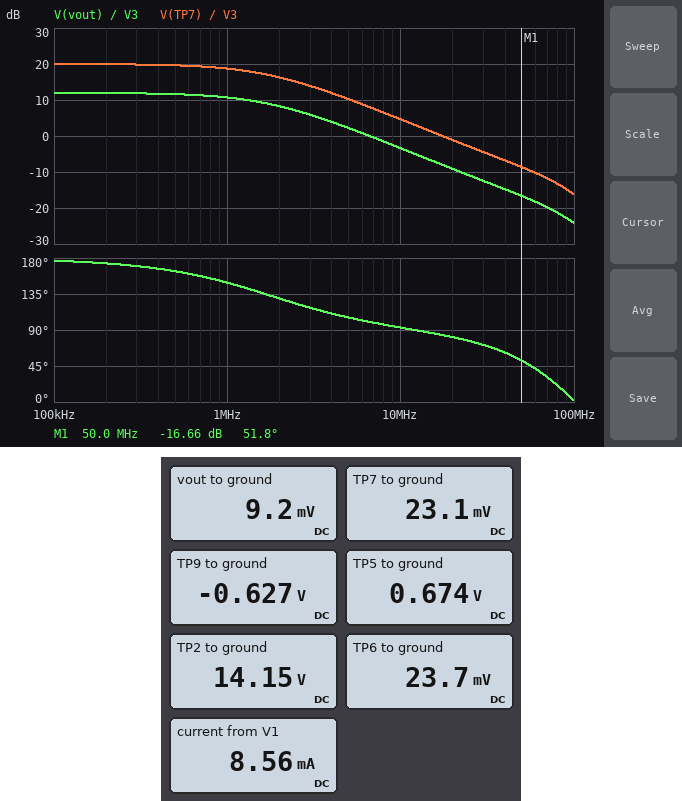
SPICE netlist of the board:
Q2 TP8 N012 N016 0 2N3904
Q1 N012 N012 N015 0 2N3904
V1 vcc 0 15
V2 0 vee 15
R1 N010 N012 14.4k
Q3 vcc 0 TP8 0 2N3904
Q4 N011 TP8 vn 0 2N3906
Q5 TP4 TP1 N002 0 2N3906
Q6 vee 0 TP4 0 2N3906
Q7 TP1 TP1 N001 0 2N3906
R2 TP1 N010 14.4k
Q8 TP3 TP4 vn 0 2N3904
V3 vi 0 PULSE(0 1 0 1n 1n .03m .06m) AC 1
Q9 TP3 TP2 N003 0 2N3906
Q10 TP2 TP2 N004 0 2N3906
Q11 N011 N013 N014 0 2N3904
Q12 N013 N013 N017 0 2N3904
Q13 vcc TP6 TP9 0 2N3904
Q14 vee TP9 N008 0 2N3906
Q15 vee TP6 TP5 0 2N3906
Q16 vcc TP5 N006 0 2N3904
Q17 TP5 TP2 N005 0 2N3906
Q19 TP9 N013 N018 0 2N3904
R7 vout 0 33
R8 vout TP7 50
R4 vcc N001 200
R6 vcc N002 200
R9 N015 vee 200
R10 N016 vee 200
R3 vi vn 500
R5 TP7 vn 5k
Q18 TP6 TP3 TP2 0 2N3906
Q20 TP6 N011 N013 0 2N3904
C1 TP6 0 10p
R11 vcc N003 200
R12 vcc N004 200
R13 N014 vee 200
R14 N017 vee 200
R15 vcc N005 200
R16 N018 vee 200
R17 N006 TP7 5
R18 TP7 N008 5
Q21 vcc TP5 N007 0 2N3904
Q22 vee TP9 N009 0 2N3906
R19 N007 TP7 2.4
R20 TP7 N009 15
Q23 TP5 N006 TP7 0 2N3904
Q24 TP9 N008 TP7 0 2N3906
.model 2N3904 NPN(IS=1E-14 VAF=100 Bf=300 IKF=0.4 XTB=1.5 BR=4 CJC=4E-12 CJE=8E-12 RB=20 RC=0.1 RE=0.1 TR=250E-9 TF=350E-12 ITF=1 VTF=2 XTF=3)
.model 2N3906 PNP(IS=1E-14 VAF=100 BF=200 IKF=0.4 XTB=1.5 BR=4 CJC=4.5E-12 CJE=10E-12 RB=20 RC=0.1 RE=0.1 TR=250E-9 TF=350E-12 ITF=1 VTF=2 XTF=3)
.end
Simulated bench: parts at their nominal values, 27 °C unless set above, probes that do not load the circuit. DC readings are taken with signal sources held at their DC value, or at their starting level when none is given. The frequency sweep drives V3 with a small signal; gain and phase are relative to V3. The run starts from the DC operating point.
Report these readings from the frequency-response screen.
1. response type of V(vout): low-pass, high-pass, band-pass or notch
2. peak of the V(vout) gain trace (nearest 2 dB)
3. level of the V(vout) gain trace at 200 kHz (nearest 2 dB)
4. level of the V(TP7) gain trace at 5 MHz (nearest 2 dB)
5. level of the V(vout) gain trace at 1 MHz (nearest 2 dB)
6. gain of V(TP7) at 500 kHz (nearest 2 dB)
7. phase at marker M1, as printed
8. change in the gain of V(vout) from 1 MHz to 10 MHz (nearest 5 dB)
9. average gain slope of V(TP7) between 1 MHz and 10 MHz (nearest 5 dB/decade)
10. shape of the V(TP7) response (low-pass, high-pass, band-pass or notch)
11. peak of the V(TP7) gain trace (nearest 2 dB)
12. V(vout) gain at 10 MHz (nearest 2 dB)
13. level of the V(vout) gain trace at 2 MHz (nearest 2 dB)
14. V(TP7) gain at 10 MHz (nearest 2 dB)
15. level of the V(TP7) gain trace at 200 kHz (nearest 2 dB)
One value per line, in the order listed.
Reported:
low-pass
12 dB
12 dB
10 dB
10 dB
20 dB
51.8 deg
-15 dB
-15 dB/decade
low-pass
20 dB
-4 dB
8 dB
4 dB
20 dB
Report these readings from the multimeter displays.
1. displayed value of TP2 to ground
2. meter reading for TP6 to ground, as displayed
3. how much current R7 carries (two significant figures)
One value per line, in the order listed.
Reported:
14.15 V
23.7 mV
280 µA
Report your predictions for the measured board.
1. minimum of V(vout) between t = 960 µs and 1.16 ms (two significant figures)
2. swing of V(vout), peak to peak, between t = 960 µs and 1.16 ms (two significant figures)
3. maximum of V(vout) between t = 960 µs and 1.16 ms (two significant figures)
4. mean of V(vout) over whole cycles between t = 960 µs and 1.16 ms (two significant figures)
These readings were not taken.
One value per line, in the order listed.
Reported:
-4.0 V
4.0 V
10 mV
-2.0 V
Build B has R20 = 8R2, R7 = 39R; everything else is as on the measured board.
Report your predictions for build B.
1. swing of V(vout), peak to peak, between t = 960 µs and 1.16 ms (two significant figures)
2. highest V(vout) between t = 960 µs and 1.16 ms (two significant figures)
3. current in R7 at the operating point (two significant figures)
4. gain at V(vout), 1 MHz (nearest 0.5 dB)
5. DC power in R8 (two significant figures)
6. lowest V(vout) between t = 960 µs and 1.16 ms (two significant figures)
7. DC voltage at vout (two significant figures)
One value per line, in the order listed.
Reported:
4.4 V
11 mV
260 µA
11.5 dB
3.4 µW
-4.4 V
10 mV
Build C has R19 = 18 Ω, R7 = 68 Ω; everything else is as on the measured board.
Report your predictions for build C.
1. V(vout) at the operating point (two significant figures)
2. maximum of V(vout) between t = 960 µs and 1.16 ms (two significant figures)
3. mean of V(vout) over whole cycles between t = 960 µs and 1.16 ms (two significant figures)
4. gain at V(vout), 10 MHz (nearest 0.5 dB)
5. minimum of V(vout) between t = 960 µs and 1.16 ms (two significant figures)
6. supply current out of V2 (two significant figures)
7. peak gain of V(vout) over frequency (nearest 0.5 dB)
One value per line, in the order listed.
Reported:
13 mV
15 mV
-2.9 V
0 dB
-5.7 V
8.2 mA
15.0 dB
